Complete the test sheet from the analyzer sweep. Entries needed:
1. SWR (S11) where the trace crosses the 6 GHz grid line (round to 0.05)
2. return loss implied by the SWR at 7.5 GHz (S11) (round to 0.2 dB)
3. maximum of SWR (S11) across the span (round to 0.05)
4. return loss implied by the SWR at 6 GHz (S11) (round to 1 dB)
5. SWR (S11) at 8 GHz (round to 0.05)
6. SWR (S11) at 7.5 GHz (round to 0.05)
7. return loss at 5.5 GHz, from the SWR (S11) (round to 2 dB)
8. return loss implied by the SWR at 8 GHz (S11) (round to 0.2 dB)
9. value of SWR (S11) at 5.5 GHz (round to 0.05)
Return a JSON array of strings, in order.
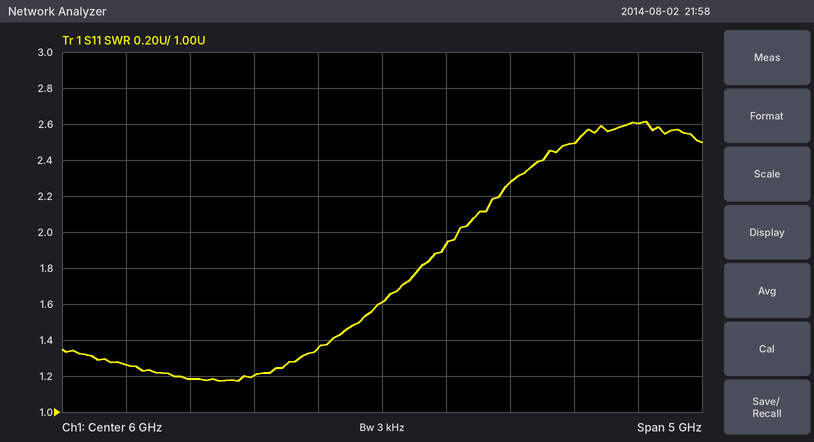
["1.60", "7.4 dB", "2.60", "13 dB", "2.60", "2.50", "16 dB", "7.0 dB", "1.35"]
